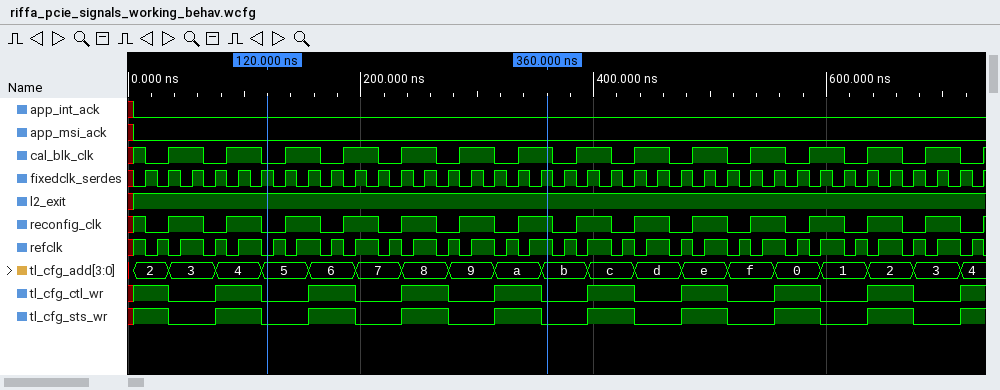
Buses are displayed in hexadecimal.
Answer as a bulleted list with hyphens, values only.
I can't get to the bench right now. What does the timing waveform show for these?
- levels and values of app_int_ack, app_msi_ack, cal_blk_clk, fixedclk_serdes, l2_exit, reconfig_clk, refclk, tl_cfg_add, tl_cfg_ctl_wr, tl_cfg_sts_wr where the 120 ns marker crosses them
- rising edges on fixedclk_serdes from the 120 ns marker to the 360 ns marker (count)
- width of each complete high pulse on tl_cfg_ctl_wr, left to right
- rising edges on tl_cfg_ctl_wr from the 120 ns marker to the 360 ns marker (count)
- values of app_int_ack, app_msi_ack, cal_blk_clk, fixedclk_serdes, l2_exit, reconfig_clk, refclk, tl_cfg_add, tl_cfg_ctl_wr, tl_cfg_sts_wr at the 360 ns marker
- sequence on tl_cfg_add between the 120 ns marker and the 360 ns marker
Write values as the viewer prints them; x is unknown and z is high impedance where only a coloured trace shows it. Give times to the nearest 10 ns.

- app_int_ack=0, app_msi_ack=0, cal_blk_clk=0, fixedclk_serdes=1, l2_exit=1, reconfig_clk=0, refclk=0, tl_cfg_add=5, tl_cfg_ctl_wr=0, tl_cfg_sts_wr=0
- 12
- 40 ns, 40 ns, 40 ns, 40 ns, 40 ns, 40 ns, 40 ns, 40 ns
- 3
- app_int_ack=0, app_msi_ack=0, cal_blk_clk=1, fixedclk_serdes=1, l2_exit=1, reconfig_clk=1, refclk=1, tl_cfg_add=b, tl_cfg_ctl_wr=0, tl_cfg_sts_wr=0
- 5, 6, 7, 8, 9, a, b
